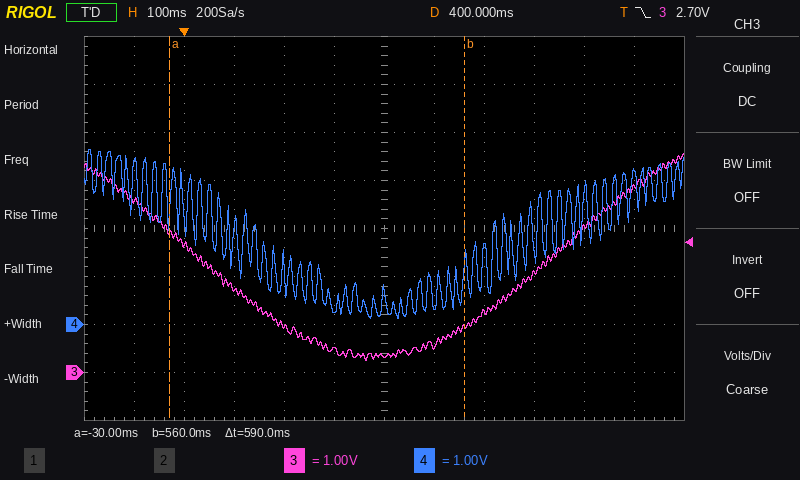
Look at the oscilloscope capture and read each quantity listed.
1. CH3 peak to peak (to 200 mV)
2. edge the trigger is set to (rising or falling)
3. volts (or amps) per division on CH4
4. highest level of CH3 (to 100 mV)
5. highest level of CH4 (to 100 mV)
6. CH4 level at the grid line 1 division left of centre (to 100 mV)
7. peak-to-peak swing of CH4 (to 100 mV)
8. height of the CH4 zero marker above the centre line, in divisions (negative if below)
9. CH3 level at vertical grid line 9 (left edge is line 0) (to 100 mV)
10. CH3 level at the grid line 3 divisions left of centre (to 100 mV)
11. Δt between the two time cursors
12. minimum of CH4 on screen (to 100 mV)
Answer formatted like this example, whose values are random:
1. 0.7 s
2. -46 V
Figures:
1. 4.4 V
2. falling
3. 1 V
4. 4.6 V
5. 3.6 V
6. 300 mV
7. 3.5 V
8. -2.0 div
9. 2.0 V
10. 1.8 V
11. 590 ms
12. 100 mV
